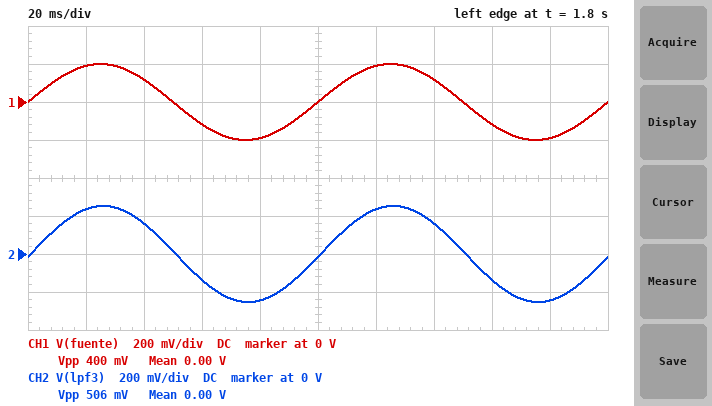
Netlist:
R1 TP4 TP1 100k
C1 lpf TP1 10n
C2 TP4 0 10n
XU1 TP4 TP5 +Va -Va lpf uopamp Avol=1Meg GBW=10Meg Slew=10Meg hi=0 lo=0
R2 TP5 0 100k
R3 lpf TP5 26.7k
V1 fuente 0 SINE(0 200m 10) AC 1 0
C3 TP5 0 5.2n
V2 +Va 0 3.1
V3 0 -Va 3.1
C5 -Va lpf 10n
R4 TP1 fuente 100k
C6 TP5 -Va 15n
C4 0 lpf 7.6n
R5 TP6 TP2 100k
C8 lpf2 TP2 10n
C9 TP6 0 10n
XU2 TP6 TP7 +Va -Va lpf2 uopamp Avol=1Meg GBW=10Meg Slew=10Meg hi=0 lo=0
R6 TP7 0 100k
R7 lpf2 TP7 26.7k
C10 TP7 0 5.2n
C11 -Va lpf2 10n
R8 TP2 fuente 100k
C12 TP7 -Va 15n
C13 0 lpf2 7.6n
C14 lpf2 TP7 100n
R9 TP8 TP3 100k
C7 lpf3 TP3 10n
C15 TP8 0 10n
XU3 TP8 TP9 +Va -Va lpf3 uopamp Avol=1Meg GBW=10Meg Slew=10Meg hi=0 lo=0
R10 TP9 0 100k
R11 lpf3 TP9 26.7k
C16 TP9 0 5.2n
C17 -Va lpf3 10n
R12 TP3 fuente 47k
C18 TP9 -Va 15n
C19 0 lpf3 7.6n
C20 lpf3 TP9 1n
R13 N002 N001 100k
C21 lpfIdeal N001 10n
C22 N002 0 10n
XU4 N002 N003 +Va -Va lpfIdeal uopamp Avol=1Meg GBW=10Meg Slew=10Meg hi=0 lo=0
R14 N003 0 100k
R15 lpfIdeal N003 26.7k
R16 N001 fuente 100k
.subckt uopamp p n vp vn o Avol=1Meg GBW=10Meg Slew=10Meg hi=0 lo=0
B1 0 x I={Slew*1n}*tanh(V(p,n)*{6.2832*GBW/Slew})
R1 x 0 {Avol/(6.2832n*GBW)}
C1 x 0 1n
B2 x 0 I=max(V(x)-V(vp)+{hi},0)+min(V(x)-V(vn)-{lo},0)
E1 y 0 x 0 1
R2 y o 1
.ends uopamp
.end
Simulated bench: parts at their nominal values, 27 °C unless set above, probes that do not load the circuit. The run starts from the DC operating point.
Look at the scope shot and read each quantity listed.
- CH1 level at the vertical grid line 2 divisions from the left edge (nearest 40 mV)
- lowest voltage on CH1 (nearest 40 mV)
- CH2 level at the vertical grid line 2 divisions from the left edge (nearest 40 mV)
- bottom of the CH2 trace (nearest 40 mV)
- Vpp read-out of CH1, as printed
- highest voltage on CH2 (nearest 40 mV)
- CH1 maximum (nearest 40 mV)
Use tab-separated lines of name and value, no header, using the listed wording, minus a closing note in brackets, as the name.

CH1 level at the vertical grid line 2 divisions from the left edge	120 mV
lowest voltage on CH1	-200 mV
CH2 level at the vertical grid line 2 divisions from the left edge	160 mV
bottom of the CH2 trace	-240 mV
Vpp read-out of CH1, as printed	400 mV
highest voltage on CH2	240 mV
CH1 maximum	200 mV
